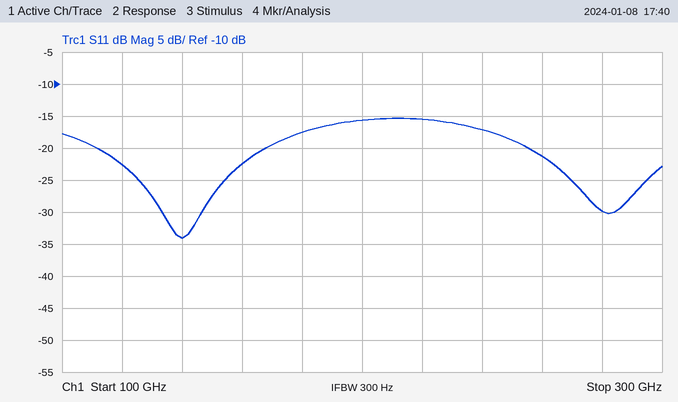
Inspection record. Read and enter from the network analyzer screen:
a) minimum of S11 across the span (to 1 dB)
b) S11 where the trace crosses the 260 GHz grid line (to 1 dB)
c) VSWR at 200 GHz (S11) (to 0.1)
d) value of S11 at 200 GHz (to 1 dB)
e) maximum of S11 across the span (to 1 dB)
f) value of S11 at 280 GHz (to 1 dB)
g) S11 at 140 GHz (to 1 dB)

-34 dB
-21 dB
1.4
-16 dB
-15 dB
-30 dB
-34 dB
